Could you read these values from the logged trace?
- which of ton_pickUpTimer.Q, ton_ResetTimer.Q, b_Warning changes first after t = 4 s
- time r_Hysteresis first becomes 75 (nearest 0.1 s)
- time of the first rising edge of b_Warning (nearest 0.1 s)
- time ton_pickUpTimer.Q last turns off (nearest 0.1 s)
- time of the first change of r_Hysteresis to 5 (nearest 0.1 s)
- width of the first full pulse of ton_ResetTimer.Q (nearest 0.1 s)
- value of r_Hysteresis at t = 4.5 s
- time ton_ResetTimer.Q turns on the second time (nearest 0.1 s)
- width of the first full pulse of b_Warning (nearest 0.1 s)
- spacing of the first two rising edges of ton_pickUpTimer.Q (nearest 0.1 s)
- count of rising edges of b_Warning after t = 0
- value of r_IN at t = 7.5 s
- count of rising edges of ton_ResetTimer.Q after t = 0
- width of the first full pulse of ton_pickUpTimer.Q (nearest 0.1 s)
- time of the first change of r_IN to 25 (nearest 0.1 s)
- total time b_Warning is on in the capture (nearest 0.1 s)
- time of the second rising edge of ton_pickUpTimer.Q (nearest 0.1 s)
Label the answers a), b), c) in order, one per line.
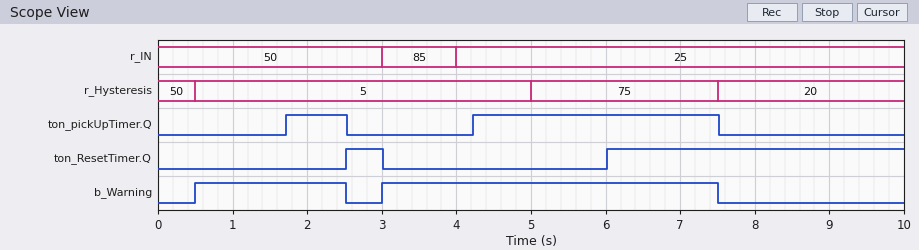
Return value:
a) ton_pickUpTimer.Q
b) 5.0 s
c) 0.5 s
d) 7.5 s
e) 0.5 s
f) 0.5 s
g) 5
h) 6.0 s
i) 2.0 s
j) 2.5 s
k) 2
l) 25
m) 2
n) 0.8 s
o) 4.0 s
p) 6.5 s
q) 4.2 s
